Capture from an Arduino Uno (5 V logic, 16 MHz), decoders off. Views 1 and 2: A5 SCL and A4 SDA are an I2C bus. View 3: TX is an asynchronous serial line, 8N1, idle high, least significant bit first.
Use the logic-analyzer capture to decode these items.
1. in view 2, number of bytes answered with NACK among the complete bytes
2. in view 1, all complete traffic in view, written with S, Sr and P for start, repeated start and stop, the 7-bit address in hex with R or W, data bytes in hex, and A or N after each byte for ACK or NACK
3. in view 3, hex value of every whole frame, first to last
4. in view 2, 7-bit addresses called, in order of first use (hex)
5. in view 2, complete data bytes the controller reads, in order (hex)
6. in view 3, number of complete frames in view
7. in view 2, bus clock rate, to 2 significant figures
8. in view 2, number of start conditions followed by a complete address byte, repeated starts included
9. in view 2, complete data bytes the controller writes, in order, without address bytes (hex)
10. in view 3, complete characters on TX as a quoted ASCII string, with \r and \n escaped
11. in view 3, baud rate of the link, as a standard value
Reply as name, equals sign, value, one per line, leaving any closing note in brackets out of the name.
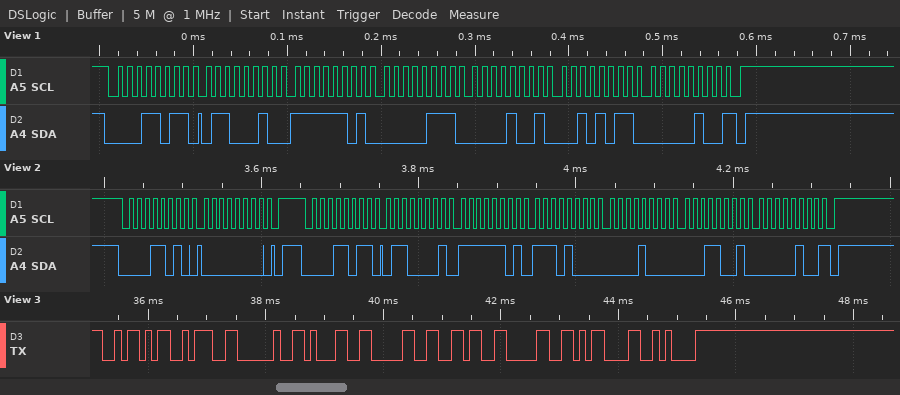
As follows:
in view 2, number of bytes answered with NACK among the complete bytes = 1
in view 1, all complete traffic in view, written with S, Sr and P for start, repeated start and stop, the 7-bit address in hex with R or W, data bytes in hex, and A or N after each byte for ACK or NACK = S 0DR A 62 A FD A 07 A 09 A 2B A 04 N P
in view 3, hex value of every whole frame, first to last = 5A 3A 20 31 30 36 30 0D 0A
in view 2, 7-bit addresses called, in order of first use = 0x0D
in view 2, complete data bytes the controller reads, in order = 61 FD E8 08 19 04
in view 3, number of complete frames in view = 9
in view 2, bus clock rate, to 2 significant figures = 100 kHz
in view 2, number of start conditions followed by a complete address byte, repeated starts included = 2
in view 2, complete data bytes the controller writes, in order, without address bytes = 00
in view 3, complete characters on TX as a quoted ASCII string, with \r and \n escaped = "Z: 1060\r\n"
in view 3, baud rate of the link, as a standard value = 9600 baud
